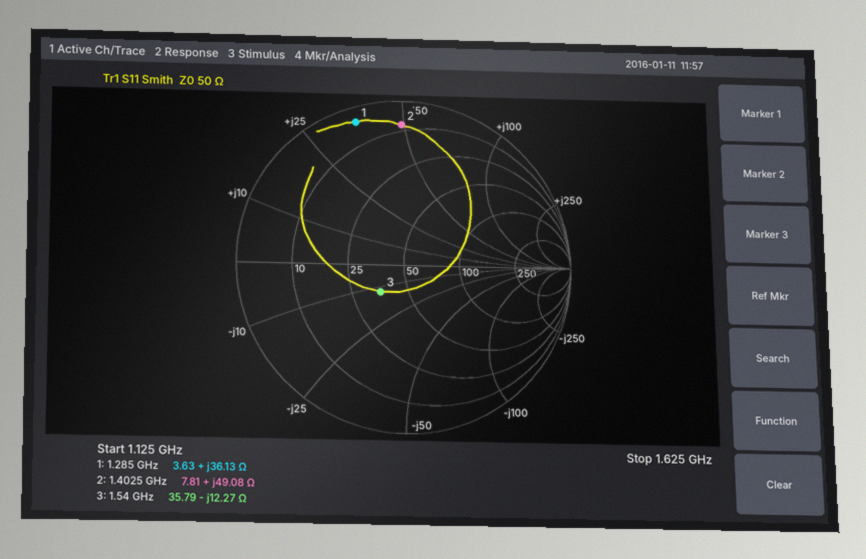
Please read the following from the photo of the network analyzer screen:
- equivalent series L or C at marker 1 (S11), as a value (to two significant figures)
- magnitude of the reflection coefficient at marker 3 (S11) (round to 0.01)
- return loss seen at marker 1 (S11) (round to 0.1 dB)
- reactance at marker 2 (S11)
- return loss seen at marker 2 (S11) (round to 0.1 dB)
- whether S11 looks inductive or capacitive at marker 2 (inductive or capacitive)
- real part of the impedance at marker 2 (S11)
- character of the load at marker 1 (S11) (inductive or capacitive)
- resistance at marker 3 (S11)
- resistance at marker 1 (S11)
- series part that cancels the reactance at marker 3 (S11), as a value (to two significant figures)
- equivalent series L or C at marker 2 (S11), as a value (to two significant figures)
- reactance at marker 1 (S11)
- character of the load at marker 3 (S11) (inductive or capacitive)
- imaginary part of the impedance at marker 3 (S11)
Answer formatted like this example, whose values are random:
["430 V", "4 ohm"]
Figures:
["4.5 nH", "0.22", "0.8 dB", "+49.08 Ω", "1.4 dB", "inductive", "7.81 Ω", "inductive", "35.79 Ω", "3.63 Ω", "1.3 nH", "5.6 nH", "+36.13 Ω", "capacitive", "-12.27 Ω"]
